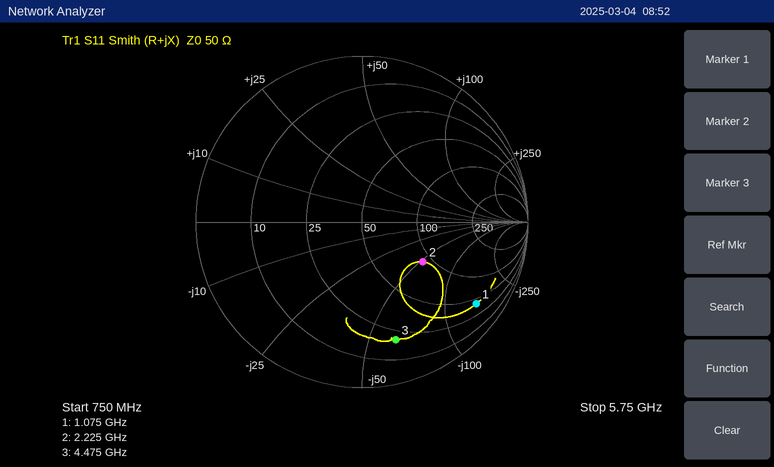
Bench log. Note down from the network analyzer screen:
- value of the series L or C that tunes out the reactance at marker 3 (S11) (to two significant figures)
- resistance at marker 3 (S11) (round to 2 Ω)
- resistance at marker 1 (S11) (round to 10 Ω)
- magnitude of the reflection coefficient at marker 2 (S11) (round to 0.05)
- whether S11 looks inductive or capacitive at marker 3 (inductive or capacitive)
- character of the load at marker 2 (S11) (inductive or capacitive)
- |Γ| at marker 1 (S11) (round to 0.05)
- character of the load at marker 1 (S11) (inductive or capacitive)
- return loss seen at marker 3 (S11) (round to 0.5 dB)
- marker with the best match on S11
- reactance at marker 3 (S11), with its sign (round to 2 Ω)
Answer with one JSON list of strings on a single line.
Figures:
["2.2 nH", "20 Ω", "40 Ω", "0.45", "capacitive", "capacitive", "0.85", "capacitive", "2.5 dB", "marker 2", "-62 Ω"]
